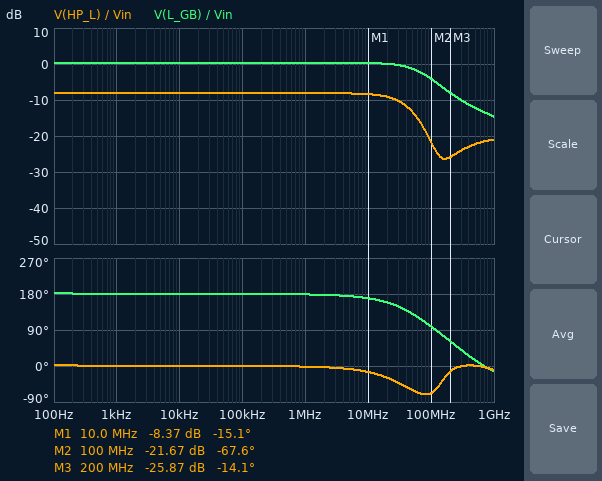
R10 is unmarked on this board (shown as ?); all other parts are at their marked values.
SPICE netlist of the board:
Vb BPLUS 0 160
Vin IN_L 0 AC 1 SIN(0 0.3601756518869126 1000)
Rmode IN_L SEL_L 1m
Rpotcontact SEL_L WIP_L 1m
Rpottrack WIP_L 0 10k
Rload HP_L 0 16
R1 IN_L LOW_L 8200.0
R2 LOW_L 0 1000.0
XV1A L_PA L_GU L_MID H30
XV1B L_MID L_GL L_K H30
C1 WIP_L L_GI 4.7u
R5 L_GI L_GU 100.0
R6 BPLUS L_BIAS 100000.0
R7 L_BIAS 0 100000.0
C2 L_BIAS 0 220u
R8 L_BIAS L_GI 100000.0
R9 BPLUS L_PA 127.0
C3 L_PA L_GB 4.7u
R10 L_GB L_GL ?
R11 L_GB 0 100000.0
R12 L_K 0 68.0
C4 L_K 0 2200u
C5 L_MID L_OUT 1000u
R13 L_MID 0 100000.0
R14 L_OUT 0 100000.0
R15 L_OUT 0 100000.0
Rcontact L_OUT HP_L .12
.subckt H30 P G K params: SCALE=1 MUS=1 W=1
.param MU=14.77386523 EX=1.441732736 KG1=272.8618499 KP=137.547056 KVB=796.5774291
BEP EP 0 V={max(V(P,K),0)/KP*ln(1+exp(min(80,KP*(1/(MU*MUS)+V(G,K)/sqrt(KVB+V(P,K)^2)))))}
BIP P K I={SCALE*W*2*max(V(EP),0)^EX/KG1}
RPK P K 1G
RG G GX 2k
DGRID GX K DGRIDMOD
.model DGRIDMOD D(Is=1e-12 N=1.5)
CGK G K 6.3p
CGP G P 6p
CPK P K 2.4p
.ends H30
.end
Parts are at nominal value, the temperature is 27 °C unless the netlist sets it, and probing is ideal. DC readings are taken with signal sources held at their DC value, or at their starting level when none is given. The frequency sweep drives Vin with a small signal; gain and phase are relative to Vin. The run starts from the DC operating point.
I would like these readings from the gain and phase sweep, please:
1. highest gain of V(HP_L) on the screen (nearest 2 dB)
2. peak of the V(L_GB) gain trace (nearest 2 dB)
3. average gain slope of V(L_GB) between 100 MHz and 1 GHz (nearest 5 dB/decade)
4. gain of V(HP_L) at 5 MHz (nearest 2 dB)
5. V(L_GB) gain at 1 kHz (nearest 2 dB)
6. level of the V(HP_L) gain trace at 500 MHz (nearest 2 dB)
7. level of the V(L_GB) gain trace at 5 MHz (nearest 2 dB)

-8 dB
0 dB
-10 dB/decade
-8 dB
0 dB
-22 dB
0 dB
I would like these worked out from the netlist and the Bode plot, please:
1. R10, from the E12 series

220 Ω
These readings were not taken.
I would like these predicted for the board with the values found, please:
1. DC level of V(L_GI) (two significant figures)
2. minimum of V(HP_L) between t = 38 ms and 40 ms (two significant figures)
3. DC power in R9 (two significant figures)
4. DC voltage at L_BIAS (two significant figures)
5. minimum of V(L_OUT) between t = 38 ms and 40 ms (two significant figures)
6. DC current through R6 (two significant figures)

80 V
-140 mV
180 mW
80 V
-140 mV
800 µA
